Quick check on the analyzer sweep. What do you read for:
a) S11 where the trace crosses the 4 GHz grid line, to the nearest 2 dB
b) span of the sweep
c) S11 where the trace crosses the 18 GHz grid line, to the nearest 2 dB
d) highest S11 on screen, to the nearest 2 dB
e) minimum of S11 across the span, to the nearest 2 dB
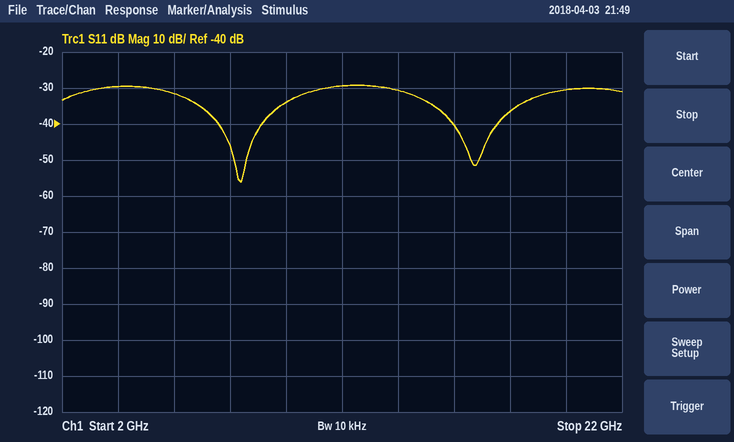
-30 dB
20 GHz
-36 dB
-30 dB
-56 dB
